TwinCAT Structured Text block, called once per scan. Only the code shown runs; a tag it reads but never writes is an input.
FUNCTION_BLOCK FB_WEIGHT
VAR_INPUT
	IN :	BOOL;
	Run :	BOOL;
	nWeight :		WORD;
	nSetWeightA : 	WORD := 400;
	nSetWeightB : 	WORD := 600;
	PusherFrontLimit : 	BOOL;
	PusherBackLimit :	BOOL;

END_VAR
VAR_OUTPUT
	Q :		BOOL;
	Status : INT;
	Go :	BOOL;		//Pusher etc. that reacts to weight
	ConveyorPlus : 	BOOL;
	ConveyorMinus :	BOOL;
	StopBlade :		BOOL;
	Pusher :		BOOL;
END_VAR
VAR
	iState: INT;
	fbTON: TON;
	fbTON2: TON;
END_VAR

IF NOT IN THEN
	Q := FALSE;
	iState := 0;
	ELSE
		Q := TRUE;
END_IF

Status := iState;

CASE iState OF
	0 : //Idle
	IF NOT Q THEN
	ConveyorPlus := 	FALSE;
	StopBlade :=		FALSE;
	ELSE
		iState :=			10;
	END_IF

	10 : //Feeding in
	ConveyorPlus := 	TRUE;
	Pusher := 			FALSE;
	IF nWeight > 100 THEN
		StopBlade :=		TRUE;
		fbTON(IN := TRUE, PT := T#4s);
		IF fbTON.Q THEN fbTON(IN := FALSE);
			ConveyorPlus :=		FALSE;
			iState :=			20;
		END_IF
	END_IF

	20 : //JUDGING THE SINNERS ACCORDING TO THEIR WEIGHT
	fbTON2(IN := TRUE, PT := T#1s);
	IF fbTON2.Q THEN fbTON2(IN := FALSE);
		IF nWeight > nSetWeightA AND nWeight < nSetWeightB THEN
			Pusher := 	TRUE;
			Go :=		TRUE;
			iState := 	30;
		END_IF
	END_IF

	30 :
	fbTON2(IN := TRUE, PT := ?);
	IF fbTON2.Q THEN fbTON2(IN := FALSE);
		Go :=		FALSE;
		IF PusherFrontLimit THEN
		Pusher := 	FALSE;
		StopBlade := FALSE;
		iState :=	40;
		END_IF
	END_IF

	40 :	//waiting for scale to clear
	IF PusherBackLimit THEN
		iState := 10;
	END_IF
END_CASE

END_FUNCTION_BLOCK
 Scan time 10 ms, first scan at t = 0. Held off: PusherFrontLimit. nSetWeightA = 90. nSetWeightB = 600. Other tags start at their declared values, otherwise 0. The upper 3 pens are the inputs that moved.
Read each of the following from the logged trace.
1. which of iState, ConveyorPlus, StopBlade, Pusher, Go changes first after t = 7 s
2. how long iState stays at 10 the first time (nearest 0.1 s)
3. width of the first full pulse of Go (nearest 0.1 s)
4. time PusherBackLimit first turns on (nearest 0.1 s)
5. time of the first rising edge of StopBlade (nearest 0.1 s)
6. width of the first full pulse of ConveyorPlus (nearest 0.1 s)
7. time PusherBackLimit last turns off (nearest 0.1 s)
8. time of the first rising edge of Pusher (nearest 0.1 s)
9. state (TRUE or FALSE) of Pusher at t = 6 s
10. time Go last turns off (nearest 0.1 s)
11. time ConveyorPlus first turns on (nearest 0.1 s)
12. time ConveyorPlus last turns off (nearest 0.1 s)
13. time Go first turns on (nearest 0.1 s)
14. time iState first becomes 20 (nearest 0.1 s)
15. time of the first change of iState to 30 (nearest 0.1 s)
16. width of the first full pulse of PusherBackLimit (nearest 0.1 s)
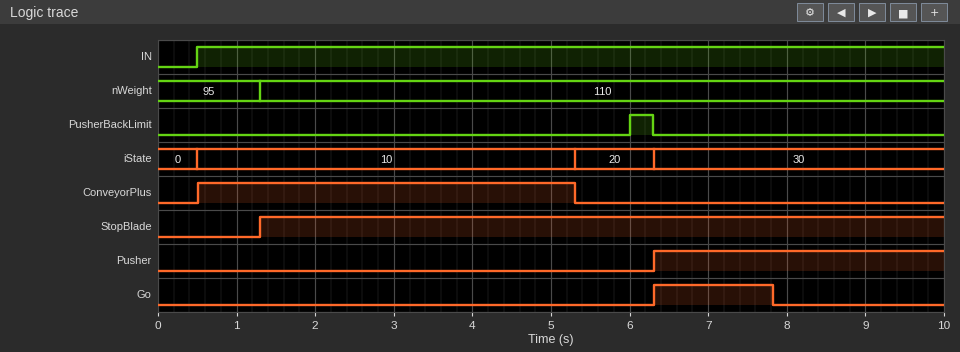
Go
4.8 s
1.5 s
6.0 s
1.3 s
4.8 s
6.3 s
6.3 s
FALSE
7.8 s
0.5 s
5.3 s
6.3 s
5.3 s
6.3 s
0.3 s
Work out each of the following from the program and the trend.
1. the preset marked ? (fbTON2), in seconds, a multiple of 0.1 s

1.5 s
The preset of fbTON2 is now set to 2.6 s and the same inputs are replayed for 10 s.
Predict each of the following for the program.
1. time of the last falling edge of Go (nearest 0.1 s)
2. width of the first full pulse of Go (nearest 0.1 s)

8.9 s
2.6 s
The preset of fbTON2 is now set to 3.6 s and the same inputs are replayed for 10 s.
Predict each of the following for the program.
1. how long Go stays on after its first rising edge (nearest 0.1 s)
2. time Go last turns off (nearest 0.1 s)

3.6 s
9.9 s
